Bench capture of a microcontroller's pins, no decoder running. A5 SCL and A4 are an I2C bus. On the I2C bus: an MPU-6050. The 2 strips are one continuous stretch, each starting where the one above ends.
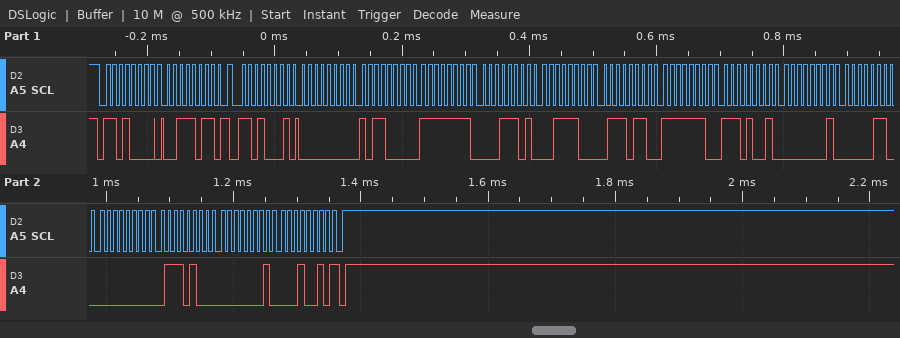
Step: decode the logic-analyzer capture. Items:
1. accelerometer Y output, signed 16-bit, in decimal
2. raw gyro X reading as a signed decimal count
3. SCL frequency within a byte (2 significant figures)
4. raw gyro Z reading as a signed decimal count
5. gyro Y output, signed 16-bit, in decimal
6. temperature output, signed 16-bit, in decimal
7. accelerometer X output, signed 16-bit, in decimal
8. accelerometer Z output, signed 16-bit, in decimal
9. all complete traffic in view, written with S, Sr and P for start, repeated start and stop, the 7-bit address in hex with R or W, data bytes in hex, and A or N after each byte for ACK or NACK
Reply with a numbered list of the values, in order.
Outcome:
1. -227
2. 262
3. 100 kHz
4. 274
5. 116
6. -279
7. 176
8. 15478
9. S 68W A 3B A Sr 68R A 00 A B0 A FF A 1D A 3C A 76 A FE A E9 A 01 A 06 A 00 A 74 A 01 A 12 N P
